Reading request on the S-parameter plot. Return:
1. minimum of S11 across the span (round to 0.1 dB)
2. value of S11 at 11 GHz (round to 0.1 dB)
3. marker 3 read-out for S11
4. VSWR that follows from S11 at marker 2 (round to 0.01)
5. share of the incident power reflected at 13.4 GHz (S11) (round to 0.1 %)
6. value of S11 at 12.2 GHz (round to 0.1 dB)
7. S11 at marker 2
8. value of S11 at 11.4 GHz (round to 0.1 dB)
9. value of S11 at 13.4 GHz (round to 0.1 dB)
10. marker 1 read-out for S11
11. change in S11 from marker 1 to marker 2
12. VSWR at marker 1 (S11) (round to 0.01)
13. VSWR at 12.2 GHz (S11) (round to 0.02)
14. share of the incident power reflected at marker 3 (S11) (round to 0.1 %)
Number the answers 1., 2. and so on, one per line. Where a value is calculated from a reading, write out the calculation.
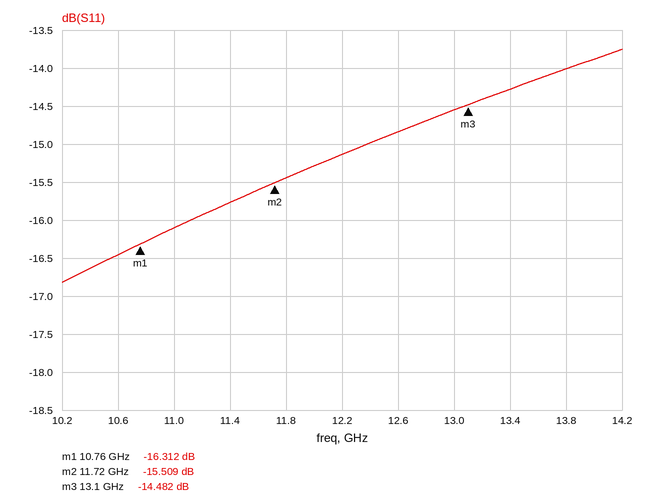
1. -16.8 dB
2. -16.1 dB
3. -14.482 dB
4. (1 + 0.1677)/(1 − 0.1677) ≈ 1.40
5. 10^(-14.3/10) ≈ 3.7 %
6. -15.1 dB
7. -15.509 dB
8. -15.8 dB
9. -14.3 dB
10. -16.312 dB
11. -15.509 − (-16.312) = 0.803 dB
12. (1 + 0.1529)/(1 − 0.1529) ≈ 1.36
13. |Γ| = 10^(-15.1/20) = 0.1758; VSWR = (1 + 0.1758)/(1 − 0.1758) ≈ 1.43, so 1.42 to the nearest 0.02
14. 10^(-14.482/10) ≈ 3.6 %
